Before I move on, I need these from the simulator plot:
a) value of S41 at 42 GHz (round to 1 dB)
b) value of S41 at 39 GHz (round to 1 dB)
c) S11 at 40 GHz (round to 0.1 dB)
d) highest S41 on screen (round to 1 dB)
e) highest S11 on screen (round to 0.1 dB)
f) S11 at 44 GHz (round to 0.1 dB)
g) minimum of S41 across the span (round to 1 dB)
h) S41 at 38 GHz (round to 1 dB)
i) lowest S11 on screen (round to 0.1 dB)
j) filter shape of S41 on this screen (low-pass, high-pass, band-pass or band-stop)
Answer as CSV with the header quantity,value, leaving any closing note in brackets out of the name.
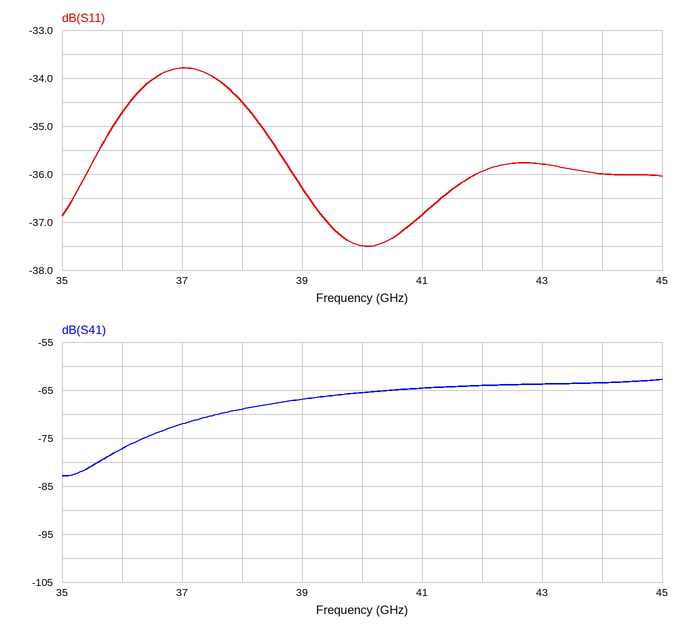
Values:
quantity,value
value of S41 at 42 GHz,-64 dB
value of S41 at 39 GHz,-67 dB
S11 at 40 GHz,-37.5 dB
highest S41 on screen,-63 dB
highest S11 on screen,-33.8 dB
S11 at 44 GHz,-36.0 dB
minimum of S41 across the span,-83 dB
S41 at 38 GHz,-69 dB
lowest S11 on screen,-37.5 dB
filter shape of S41 on this screen,high-pass
